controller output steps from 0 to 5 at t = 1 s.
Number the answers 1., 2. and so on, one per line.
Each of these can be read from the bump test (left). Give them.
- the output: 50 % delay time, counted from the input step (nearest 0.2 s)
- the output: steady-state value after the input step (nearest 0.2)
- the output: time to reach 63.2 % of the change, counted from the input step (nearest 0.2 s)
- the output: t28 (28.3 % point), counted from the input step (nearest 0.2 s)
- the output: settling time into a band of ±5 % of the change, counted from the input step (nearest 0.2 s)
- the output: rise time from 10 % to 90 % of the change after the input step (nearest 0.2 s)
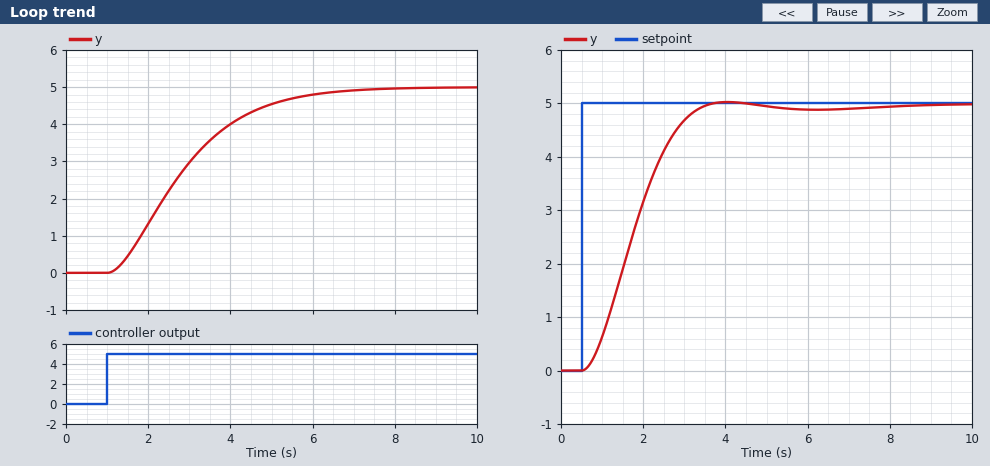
1. 1.6 s
2. 5.0
3. 2.2 s
4. 1.0 s
5. 4.8 s
6. 3.4 s
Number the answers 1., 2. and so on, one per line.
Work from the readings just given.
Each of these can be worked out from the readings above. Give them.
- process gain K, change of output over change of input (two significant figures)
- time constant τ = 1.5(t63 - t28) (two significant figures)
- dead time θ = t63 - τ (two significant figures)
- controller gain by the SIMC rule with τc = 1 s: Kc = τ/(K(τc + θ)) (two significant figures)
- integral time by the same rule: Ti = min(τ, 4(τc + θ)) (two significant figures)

1. 1.0
2. 1.8 s
3. 0.40 s
4. 1.3
5. 1.8 s
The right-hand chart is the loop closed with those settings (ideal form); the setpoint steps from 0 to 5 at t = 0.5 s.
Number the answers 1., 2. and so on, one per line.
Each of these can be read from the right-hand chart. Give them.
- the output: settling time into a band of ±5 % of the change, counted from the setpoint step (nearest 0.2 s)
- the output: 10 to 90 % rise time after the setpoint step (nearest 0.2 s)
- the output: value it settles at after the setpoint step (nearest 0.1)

1. 2.6 s
2. 1.8 s
3. 5.0
